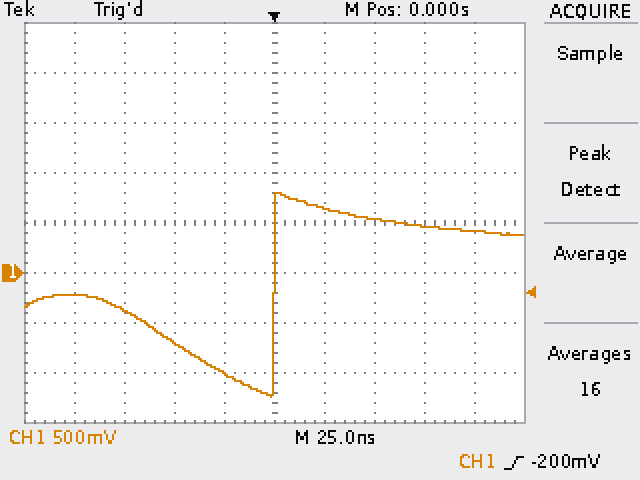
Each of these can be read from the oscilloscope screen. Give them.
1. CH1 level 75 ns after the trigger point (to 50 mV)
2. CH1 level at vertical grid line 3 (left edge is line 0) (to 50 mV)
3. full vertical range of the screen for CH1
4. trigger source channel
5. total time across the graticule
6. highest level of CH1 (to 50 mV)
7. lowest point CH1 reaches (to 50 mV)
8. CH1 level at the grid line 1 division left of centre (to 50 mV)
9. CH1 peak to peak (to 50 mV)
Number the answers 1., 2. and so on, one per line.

1. 450 mV
2. -700 mV
3. 4 V
4. CH1
5. 250 ns
6. 800 mV
7. -1.25 V
8. -1.00 V
9. 2.05 V
